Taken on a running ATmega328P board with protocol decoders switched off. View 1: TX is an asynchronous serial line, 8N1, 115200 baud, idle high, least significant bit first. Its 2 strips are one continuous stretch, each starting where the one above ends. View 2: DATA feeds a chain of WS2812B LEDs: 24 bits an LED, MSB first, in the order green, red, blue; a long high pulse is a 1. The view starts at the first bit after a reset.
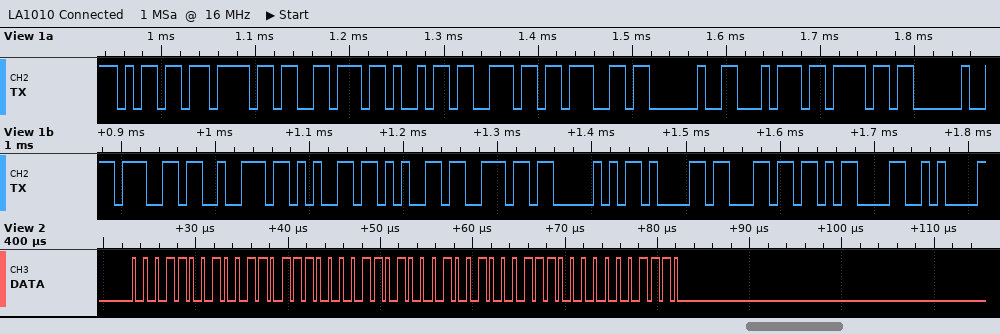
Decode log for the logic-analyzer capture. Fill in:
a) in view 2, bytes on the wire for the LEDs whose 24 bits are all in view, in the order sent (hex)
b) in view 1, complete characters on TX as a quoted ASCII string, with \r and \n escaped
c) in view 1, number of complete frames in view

19 37 0D 12 38 0E
"moving to greenPal\r\n"
20
